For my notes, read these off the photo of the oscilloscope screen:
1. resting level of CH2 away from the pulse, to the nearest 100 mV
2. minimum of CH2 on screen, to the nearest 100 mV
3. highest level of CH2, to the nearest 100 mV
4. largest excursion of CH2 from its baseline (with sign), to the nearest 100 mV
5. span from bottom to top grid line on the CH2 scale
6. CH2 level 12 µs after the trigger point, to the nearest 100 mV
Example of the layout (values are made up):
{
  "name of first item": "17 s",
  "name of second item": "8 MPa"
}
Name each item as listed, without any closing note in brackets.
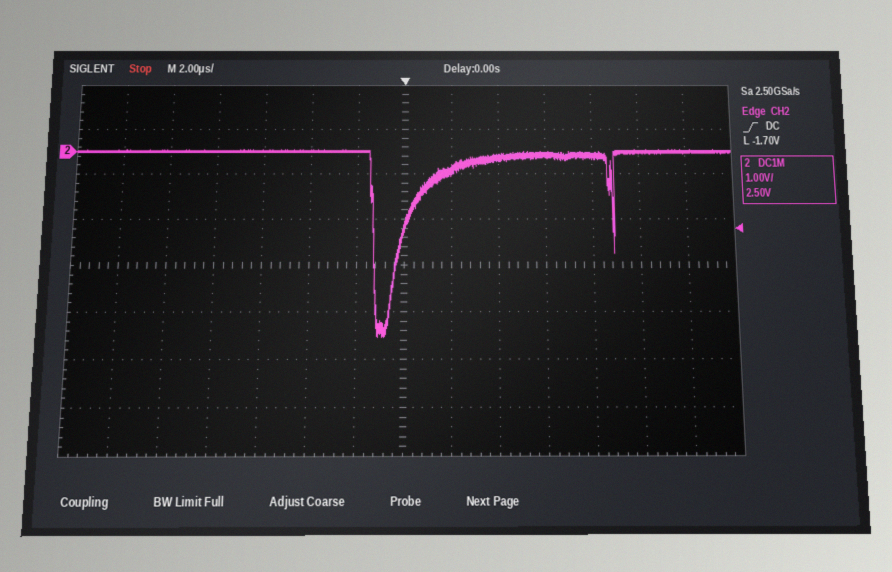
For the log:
{
  "resting level of CH2 away from the pulse, to the nearest 100 mV": "0.0 V",
  "minimum of CH2 on screen, to the nearest 100 mV": "-4.0 V",
  "highest level of CH2, to the nearest 100 mV": "0.0 V",
  "largest excursion of CH2 from its baseline (with sign), to the nearest 100 mV": "-4.0 V",
  "span from bottom to top grid line on the CH2 scale": "8 V",
  "CH2 level 12 µs after the trigger point, to the nearest 100 mV": "0.0 V"
}
